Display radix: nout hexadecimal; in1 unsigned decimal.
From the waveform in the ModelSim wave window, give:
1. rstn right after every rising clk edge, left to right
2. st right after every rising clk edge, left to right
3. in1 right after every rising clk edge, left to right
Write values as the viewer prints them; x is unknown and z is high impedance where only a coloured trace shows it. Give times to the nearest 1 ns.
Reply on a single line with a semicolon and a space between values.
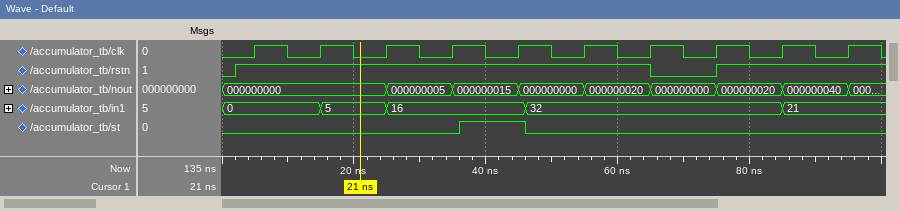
1 1 1 1 1 1 0 1 1 1; 0 0 0 0 1 0 0 0 0 0; 0, 5, 16, 16, 16, 32, 32, 32, 21, 21
